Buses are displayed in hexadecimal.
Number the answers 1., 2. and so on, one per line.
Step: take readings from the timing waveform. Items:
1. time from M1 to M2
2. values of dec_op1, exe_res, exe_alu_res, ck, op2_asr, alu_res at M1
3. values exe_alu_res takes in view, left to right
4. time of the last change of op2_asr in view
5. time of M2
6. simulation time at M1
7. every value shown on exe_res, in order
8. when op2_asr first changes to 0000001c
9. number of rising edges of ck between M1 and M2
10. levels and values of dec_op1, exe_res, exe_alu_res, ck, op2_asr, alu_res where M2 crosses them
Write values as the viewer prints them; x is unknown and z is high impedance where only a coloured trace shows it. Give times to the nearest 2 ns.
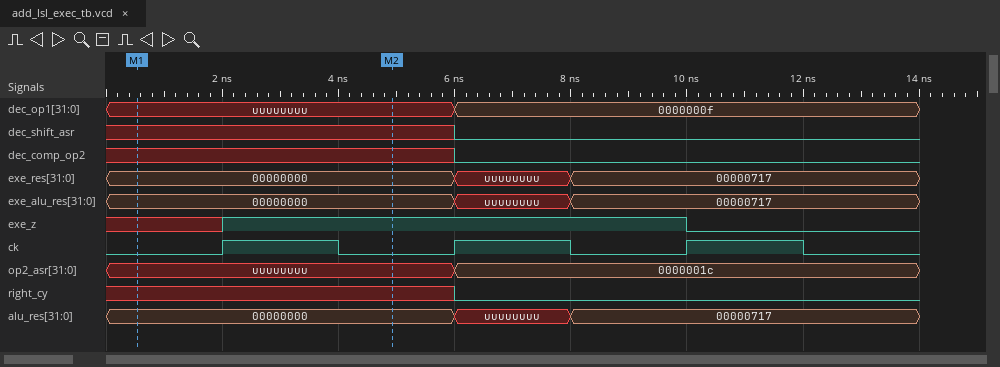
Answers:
1. 4 ns
2. dec_op1=uuuuuuuu, exe_res=00000000, exe_alu_res=00000000, ck=0, op2_asr=uuuuuuuu, alu_res=00000000
3. 00000000, uuuuuuuu, 00000717
4. 6 ns
5. 4 ns
6. 0 ns
7. 00000000, uuuuuuuu, 00000717
8. 6 ns
9. 1
10. dec_op1=uuuuuuuu, exe_res=00000000, exe_alu_res=00000000, ck=0, op2_asr=uuuuuuuu, alu_res=00000000
